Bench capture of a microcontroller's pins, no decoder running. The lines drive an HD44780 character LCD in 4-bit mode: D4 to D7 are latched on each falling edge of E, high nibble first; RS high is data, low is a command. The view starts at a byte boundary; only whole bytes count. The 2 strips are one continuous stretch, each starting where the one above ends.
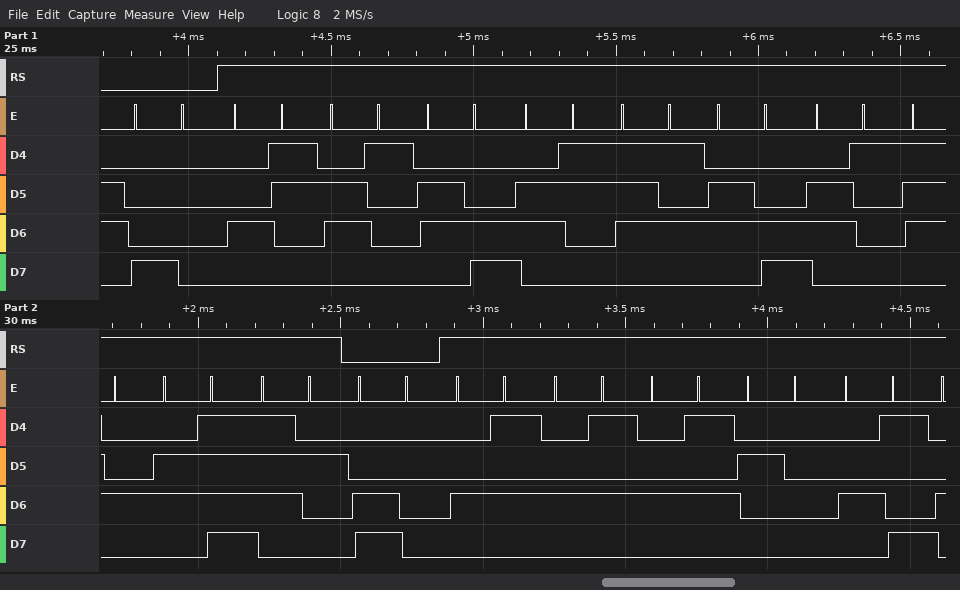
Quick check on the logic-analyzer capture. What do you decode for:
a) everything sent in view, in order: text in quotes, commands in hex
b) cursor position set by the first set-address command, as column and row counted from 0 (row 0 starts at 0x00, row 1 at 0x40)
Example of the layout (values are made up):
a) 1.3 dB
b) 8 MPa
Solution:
a) 0x80 "Calculator" 0xC0 "EEE I"
b) column 0, row 0
